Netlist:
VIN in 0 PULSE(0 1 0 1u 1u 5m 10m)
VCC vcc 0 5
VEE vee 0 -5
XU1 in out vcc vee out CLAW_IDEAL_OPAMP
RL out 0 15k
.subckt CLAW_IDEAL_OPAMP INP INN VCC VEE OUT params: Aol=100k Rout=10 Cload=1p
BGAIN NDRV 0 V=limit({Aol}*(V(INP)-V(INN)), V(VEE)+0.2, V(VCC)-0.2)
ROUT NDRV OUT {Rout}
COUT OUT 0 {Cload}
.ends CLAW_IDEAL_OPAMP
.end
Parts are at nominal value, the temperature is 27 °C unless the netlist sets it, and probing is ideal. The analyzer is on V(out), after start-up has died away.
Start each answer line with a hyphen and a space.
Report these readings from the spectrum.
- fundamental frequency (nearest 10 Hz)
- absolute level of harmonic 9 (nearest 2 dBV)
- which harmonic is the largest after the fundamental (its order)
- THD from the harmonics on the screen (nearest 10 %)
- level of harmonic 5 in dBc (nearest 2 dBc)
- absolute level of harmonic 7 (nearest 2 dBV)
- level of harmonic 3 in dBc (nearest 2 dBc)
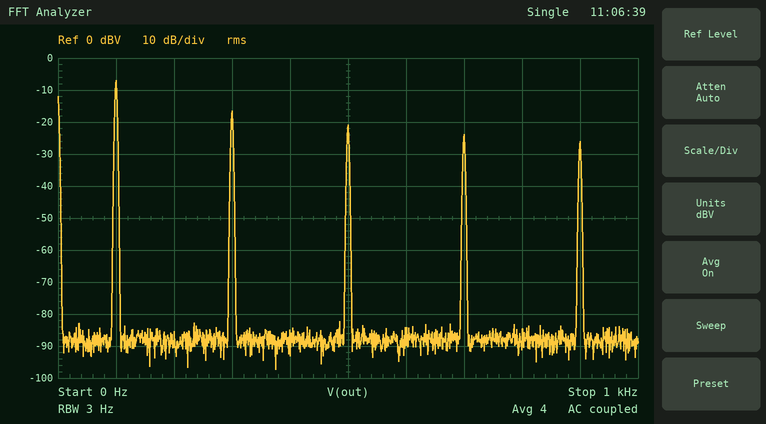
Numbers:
- 100 Hz
- -26 dBV
- 3
- 40 %
- -14 dBc
- -24 dBV
- -10 dBc
